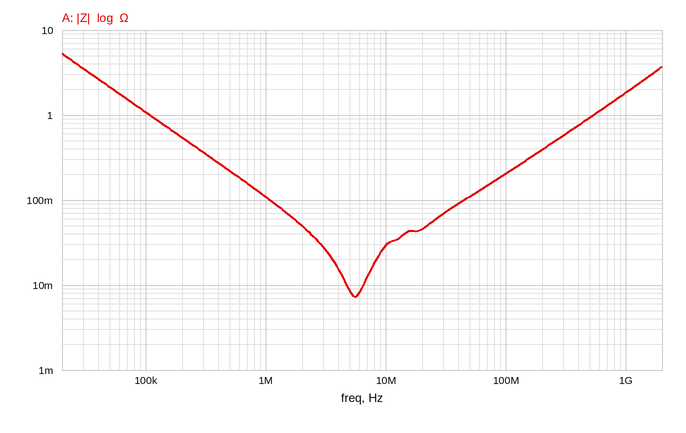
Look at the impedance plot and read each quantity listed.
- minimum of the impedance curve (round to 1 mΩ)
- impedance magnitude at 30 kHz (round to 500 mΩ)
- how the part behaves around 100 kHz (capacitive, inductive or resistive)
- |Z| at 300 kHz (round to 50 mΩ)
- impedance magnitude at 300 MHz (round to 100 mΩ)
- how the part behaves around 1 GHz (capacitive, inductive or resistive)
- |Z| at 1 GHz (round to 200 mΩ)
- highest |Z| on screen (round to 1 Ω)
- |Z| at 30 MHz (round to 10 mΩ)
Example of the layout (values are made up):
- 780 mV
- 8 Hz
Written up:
- 7 mΩ
- 3.5 Ω
- capacitive
- 350 mΩ
- 600 mΩ
- inductive
- 1.8 Ω
- 5 Ω
- 70 mΩ
